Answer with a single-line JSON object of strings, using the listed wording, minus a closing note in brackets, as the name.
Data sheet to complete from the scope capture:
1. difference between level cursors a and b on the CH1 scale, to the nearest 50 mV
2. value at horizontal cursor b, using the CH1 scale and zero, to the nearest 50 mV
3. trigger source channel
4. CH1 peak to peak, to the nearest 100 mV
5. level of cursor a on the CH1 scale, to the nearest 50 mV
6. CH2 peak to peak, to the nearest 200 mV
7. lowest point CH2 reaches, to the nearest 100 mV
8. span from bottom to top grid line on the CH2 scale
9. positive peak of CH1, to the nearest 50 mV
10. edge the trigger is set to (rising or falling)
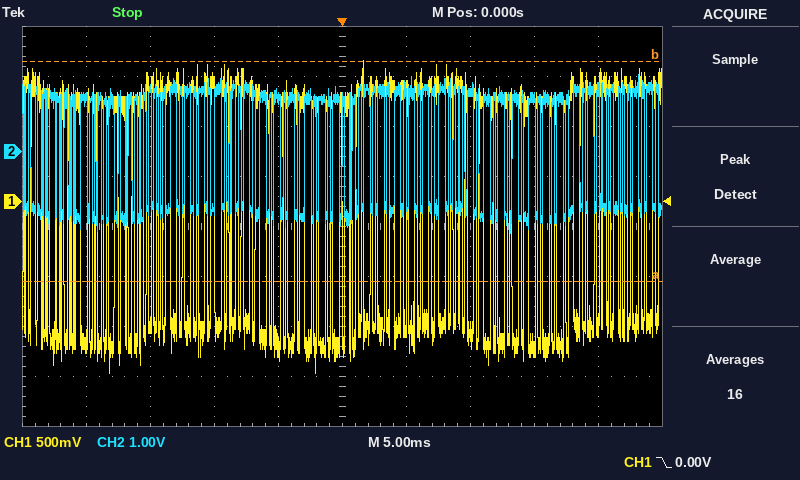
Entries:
{"difference between level cursors a and b on the CH1 scale, to the nearest 50 mV": "2.20 V", "value at horizontal cursor b, using the CH1 scale and zero, to the nearest 50 mV": "1.40 V", "trigger source channel": "CH1", "CH1 peak to peak, to the nearest 100 mV": "3.10 V", "level of cursor a on the CH1 scale, to the nearest 50 mV": "-800 mV", "CH2 peak to peak, to the nearest 200 mV": "3.2 V", "lowest point CH2 reaches, to the nearest 100 mV": "-1.6 V", "span from bottom to top grid line on the CH2 scale": "8 V", "positive peak of CH1, to the nearest 50 mV": "1.40 V", "edge the trigger is set to": "falling"}
